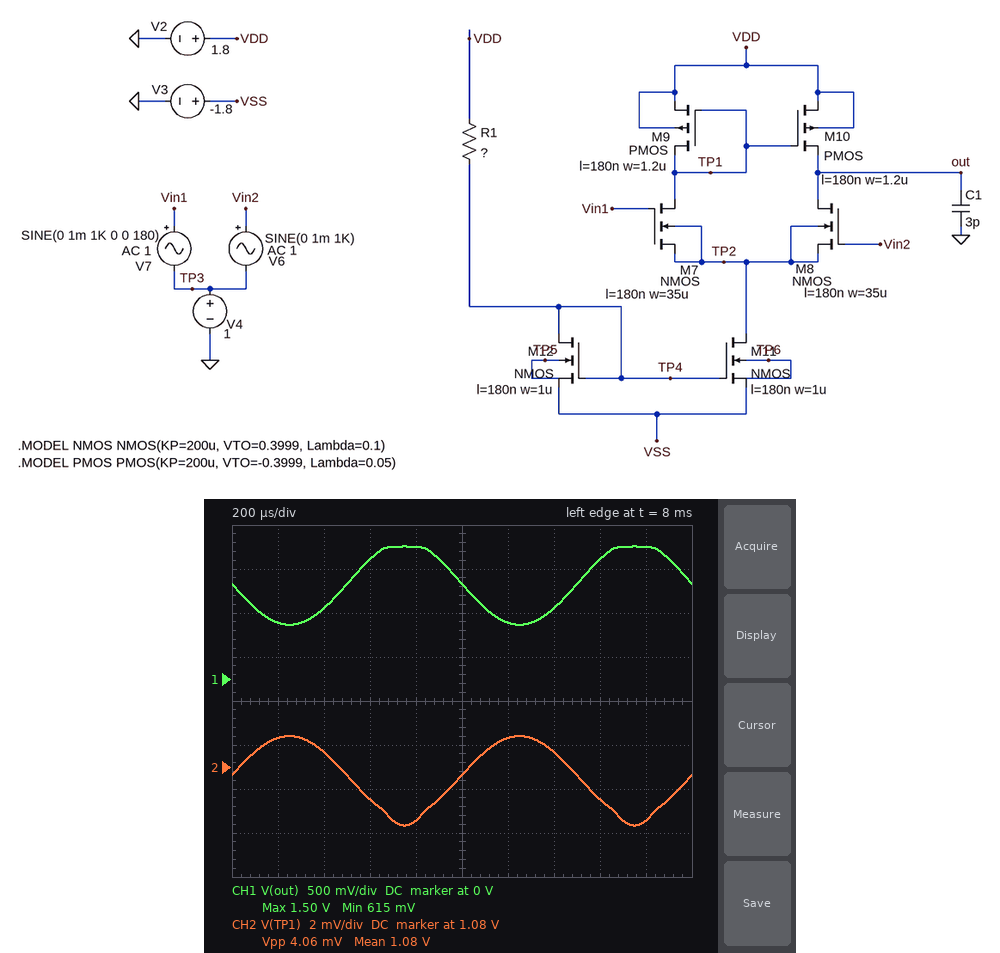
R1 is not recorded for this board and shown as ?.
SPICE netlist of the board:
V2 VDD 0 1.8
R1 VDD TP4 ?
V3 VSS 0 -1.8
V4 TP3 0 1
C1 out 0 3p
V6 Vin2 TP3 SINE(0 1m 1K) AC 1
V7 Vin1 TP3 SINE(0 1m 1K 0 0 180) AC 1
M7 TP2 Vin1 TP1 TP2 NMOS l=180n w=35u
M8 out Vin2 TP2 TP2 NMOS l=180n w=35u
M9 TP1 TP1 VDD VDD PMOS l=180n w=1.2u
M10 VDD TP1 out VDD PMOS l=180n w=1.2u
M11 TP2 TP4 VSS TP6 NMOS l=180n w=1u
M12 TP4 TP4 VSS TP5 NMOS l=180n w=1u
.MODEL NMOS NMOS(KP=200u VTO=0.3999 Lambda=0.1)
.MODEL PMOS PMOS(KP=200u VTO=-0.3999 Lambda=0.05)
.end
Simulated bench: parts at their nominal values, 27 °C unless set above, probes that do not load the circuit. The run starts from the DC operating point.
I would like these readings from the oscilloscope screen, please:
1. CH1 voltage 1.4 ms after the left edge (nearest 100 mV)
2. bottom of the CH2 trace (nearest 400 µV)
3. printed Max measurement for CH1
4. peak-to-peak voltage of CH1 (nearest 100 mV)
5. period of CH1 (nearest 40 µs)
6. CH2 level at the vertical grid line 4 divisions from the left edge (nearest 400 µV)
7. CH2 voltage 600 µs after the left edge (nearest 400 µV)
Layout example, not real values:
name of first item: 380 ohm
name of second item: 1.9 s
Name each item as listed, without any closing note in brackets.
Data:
CH1 voltage 1.4 ms after the left edge: 800 mV
bottom of the CH2 trace: 1.0772 V
printed Max measurement for CH1: 1.50 V
peak-to-peak voltage of CH1: 900 mV
period of CH1: 1.00 ms
CH2 level at the vertical grid line 4 divisions from the left edge: 1.0776 V
CH2 voltage 600 µs after the left edge: 1.0784 V
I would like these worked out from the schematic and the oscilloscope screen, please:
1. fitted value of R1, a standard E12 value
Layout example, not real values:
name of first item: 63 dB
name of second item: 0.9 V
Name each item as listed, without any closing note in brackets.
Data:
fitted value of R1, a standard E12 value: 22 kΩ
